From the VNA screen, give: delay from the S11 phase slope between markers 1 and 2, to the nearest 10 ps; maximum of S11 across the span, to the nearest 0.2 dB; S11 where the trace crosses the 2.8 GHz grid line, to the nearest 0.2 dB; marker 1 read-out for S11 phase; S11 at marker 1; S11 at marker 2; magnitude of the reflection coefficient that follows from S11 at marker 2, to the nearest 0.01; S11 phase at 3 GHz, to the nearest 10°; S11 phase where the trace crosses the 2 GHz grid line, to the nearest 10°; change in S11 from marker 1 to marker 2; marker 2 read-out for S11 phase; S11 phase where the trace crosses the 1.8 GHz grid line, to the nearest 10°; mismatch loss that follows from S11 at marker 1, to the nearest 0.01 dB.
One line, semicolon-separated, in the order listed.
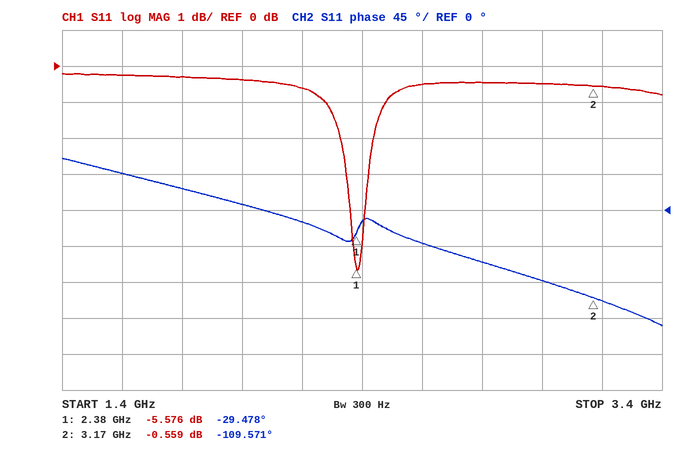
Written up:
280 ps; -0.2 dB; -0.4 dB; -29.478°; -5.576 dB; -0.559 dB; 0.94; -90°; 10°; 5.017 dB; -109.571°; 30°; 1.41 dB
